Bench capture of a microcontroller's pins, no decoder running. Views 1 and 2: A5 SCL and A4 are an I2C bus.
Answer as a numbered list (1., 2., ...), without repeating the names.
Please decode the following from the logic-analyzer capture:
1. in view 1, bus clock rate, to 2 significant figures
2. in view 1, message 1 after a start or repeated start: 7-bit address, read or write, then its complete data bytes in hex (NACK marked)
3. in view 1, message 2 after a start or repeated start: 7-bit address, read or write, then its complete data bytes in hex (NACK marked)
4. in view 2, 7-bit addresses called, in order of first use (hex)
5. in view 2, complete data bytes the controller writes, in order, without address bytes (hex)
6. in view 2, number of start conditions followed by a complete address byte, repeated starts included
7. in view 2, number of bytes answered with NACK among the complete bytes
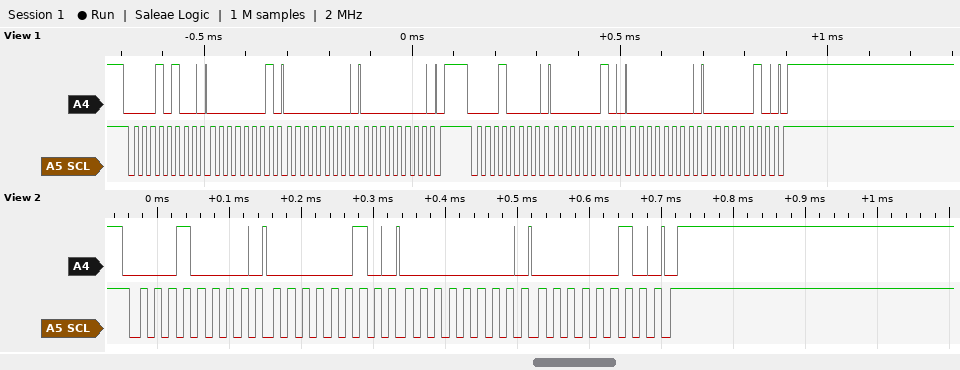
1. 50 kHz
2. 0x0A write: 01 00 00
3. 0x08 write: 02 00 02
4. 0x08
5. 02 00 02
6. 1
7. 0
